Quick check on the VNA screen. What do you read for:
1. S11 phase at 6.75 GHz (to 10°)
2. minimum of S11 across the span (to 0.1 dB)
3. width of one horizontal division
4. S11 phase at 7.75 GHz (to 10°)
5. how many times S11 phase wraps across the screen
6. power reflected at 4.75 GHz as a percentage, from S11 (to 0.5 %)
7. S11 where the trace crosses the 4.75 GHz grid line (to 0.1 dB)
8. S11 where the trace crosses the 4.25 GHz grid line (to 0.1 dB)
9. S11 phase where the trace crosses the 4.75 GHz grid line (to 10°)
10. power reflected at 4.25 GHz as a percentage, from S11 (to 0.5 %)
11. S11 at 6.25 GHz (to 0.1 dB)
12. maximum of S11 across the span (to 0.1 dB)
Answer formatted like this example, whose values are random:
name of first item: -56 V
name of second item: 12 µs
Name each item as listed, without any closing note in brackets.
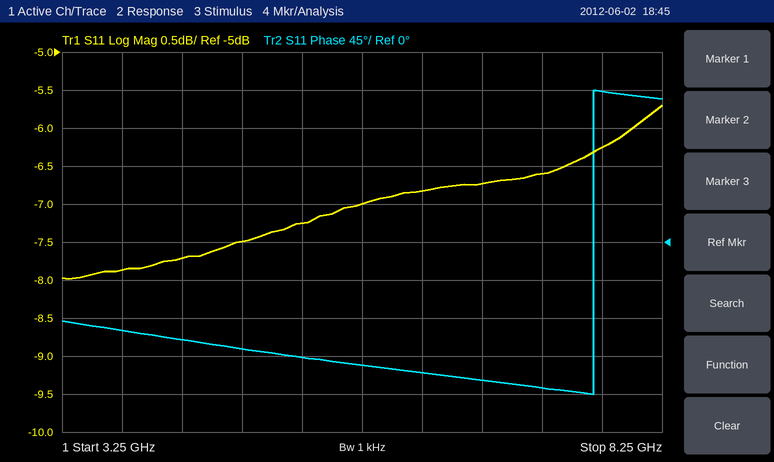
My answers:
S11 phase at 6.75 GHz: -160°
minimum of S11 across the span: -8.0 dB
width of one horizontal division: 500 MHz
S11 phase at 7.75 GHz: 180°
how many times S11 phase wraps across the screen: 1
power reflected at 4.75 GHz as a percentage, from S11: 18.0 %
S11 where the trace crosses the 4.75 GHz grid line: -7.5 dB
S11 where the trace crosses the 4.25 GHz grid line: -7.7 dB
S11 phase where the trace crosses the 4.75 GHz grid line: -130°
power reflected at 4.25 GHz as a percentage, from S11: 17.0 %
S11 at 6.25 GHz: -6.8 dB
maximum of S11 across the span: -5.7 dB
